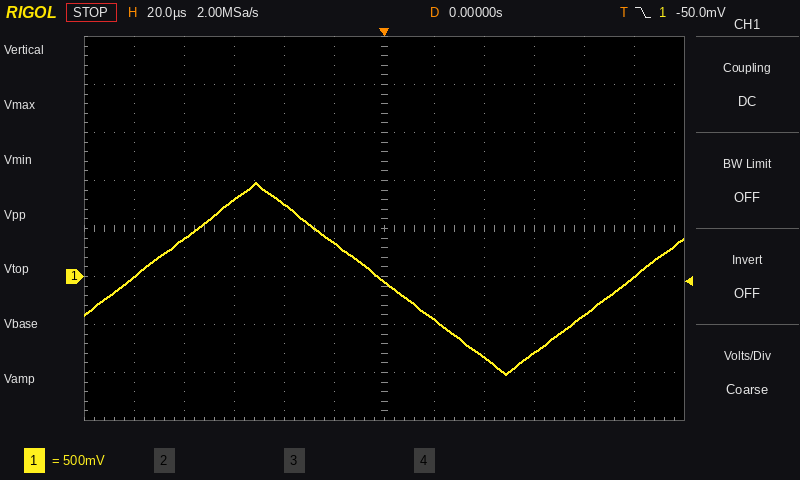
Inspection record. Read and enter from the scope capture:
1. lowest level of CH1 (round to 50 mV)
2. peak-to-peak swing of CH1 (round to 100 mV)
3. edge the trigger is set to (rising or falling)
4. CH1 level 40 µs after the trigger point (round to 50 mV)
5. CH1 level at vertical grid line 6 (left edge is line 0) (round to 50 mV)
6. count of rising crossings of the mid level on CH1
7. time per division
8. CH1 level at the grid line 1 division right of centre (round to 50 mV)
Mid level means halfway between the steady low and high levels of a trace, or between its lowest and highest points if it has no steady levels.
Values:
-1.00 V
2.00 V
falling
-850 mV
-50 mV
2
20 µs
-450 mV
